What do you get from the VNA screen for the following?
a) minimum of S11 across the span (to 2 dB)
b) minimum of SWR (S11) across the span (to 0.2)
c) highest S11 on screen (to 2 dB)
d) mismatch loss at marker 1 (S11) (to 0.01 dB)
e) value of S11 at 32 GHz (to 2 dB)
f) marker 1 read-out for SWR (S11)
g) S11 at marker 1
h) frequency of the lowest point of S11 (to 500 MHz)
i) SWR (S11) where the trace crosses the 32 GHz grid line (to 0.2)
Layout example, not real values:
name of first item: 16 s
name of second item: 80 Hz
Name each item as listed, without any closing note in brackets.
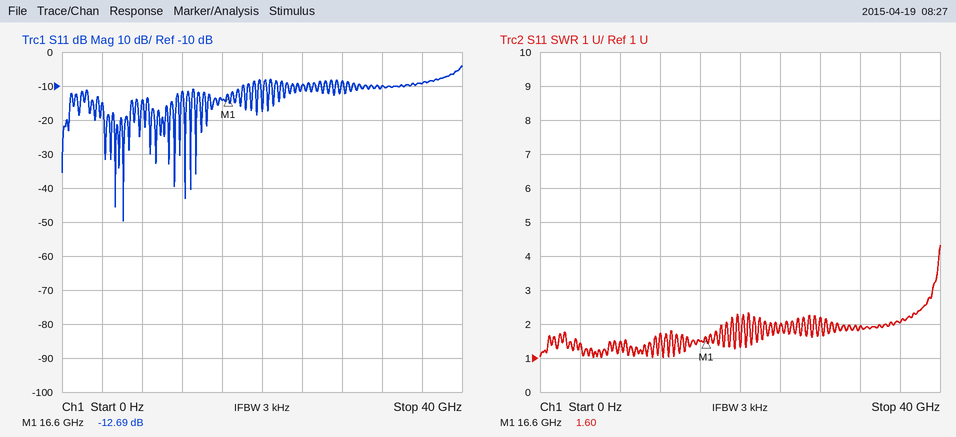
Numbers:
minimum of S11 across the span: -50 dB
minimum of SWR (S11) across the span: 1.0
highest S11 on screen: -4 dB
mismatch loss at marker 1 (S11): 0.24 dB
value of S11 at 32 GHz: -10 dB
marker 1 read-out for SWR: 1.60
S11 at marker 1: -12.69 dB
frequency of the lowest point of S11: 6.0 GHz
SWR (S11) where the trace crosses the 32 GHz grid line: 2.0
